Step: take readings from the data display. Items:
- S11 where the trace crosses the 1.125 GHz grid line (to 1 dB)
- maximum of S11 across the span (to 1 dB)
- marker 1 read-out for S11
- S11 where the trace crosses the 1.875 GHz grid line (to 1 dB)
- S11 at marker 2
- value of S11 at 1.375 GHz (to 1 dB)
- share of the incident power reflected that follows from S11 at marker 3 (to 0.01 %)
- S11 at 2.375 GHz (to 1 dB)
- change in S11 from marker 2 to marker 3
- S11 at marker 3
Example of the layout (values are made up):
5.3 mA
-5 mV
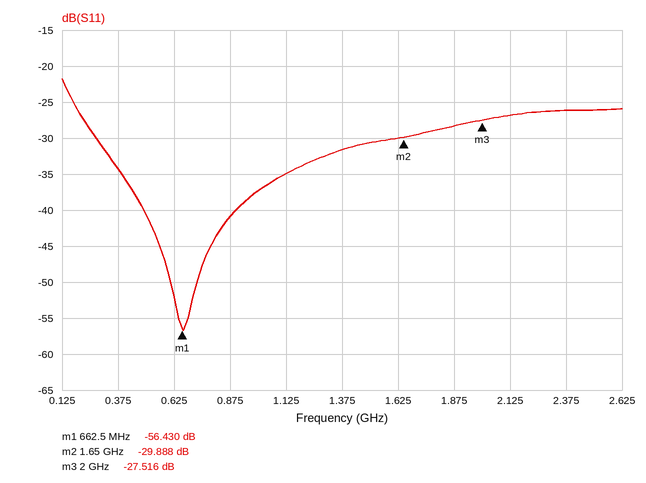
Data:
-35 dB
-22 dB
-56.430 dB
-28 dB
-29.888 dB
-32 dB
0.18 %
-26 dB
2.372 dB
-27.516 dB
